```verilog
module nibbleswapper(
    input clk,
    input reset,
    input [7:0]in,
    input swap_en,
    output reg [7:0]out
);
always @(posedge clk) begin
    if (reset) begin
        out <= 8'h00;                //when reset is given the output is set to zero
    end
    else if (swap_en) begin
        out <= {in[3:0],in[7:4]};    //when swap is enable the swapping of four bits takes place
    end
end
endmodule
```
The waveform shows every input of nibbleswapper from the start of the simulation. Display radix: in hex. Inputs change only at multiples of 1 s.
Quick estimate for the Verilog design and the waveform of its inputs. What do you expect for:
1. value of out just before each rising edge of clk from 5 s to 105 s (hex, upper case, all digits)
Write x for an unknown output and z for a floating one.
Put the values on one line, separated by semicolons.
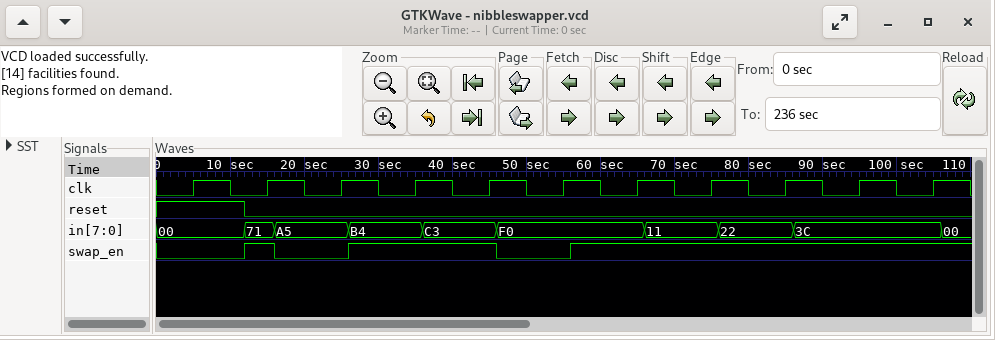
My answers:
x, 00, 17, 17, 4B, 3C, 3C, 0F, 11, 22, C3
